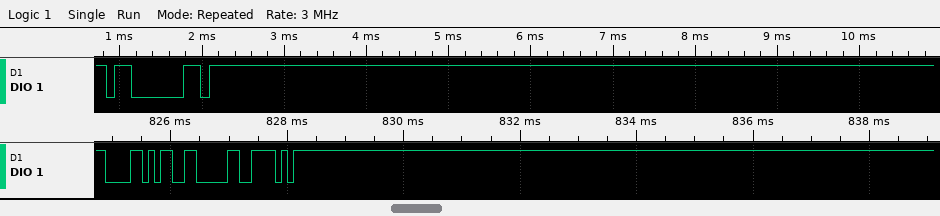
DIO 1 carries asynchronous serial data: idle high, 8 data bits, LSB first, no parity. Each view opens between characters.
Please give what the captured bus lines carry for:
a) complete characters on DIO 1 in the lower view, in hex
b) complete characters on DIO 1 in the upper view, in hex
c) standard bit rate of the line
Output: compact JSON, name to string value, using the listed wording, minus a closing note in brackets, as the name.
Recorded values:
{"complete characters on DIO 1 in the lower view, in hex": "58, 06, 5E", "complete characters on DIO 1 in the upper view, in hex": "03, FF", "standard bit rate of the line": "9600 baud"}
